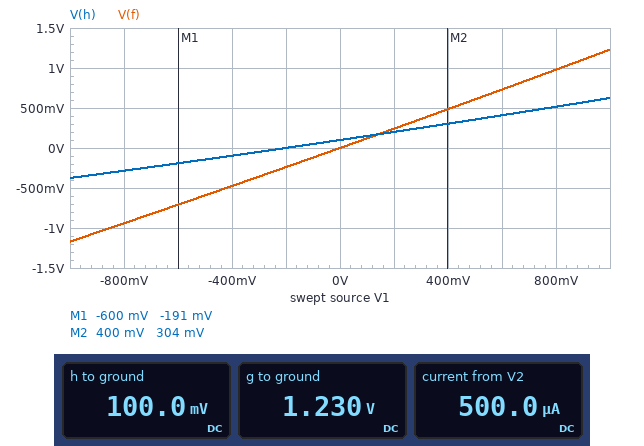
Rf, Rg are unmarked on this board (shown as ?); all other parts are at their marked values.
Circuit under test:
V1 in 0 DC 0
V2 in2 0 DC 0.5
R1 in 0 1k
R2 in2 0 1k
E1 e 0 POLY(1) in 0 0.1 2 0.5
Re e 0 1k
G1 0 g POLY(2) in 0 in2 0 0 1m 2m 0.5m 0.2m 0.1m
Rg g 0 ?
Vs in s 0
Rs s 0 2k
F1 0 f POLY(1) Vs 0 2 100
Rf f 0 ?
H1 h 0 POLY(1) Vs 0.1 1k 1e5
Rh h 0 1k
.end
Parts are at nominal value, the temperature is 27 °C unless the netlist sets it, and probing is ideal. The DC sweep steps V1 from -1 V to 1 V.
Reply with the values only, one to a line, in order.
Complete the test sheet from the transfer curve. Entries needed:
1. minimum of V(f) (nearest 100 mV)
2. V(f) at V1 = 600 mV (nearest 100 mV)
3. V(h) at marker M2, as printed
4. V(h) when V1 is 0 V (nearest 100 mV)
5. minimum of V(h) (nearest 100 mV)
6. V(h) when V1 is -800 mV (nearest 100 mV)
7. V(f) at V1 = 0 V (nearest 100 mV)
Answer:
-1.2 V
700 mV
304 mV
100 mV
-400 mV
-300 mV
0 V
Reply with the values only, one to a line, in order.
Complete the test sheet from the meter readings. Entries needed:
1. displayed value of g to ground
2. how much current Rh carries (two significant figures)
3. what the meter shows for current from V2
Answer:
1.230 V
100 µA
500.0 µA
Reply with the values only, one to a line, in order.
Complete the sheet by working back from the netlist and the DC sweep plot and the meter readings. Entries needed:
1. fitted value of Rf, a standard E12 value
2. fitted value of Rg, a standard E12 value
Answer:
1.2 kΩ
1.2 kΩ
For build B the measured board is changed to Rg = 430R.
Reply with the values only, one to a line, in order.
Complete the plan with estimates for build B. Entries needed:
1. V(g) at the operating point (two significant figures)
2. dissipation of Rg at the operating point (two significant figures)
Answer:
440 mV
450 µW
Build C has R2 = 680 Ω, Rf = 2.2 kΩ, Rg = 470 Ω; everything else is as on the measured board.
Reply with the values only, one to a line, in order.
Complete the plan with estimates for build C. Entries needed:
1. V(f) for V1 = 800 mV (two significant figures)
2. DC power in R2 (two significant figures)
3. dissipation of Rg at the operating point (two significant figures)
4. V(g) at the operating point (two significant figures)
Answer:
1.8 V
370 µW
490 µW
480 mV
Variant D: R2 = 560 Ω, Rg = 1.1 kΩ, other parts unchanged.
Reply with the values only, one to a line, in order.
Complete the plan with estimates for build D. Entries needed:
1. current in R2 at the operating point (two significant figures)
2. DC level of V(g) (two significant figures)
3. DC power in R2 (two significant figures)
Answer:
890 µA
1.1 V
450 µW
